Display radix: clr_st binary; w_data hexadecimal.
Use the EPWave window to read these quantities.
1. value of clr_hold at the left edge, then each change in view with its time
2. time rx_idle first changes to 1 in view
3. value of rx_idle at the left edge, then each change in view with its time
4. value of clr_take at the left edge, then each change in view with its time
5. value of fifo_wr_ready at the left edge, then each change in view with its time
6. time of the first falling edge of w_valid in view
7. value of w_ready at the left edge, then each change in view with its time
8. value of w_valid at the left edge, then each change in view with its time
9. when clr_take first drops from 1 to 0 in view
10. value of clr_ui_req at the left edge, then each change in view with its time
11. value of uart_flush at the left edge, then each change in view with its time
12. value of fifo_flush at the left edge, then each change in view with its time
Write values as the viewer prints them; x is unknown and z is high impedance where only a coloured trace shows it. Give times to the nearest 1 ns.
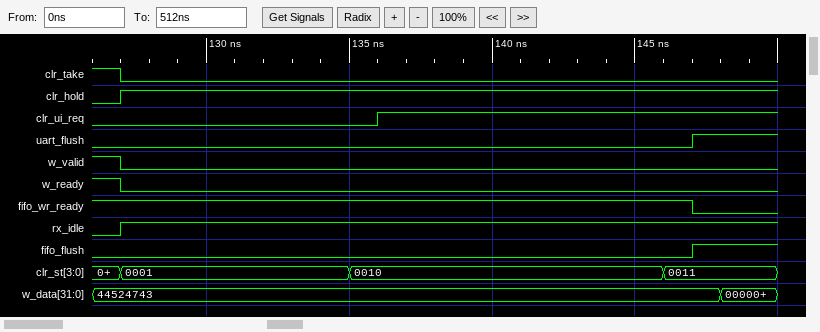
0, 1 at 127 ns
127 ns
0, 1 at 127 ns
1, 0 at 127 ns
1, 0 at 147 ns
127 ns
1, 0 at 127 ns
1, 0 at 127 ns
127 ns
0, 1 at 136 ns
0, 1 at 147 ns
0, 1 at 147 ns
